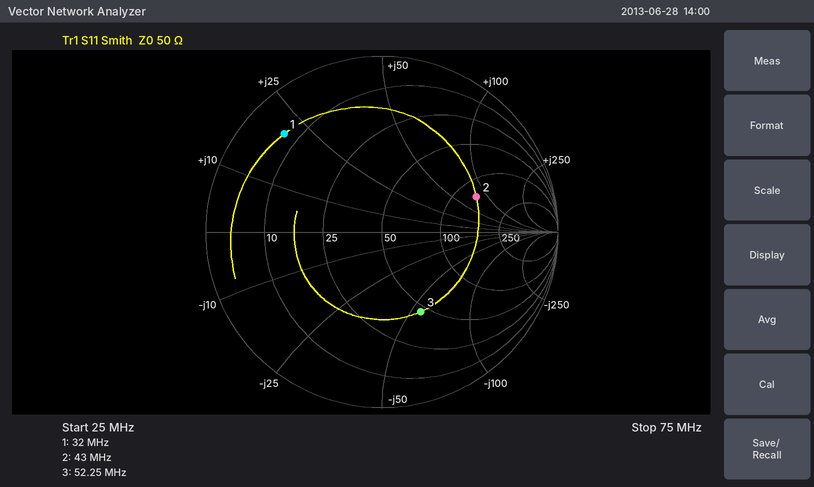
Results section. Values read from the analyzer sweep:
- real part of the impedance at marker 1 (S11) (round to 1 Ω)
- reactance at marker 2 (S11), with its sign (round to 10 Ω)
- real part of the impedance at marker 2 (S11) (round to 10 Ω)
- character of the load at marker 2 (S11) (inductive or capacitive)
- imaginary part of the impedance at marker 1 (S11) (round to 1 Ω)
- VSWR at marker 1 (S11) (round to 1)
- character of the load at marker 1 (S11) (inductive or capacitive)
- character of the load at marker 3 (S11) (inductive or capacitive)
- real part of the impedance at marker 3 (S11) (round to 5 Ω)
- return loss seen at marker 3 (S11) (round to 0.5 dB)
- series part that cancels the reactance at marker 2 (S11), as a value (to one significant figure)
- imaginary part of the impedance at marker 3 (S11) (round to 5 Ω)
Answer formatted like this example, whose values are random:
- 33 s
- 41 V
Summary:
- 7 Ω
- +80 Ω
- 130 Ω
- inductive
- +20 Ω
- 8
- inductive
- capacitive
- 45 Ω
- 6.0 dB
- 50 pF
- -55 Ω
